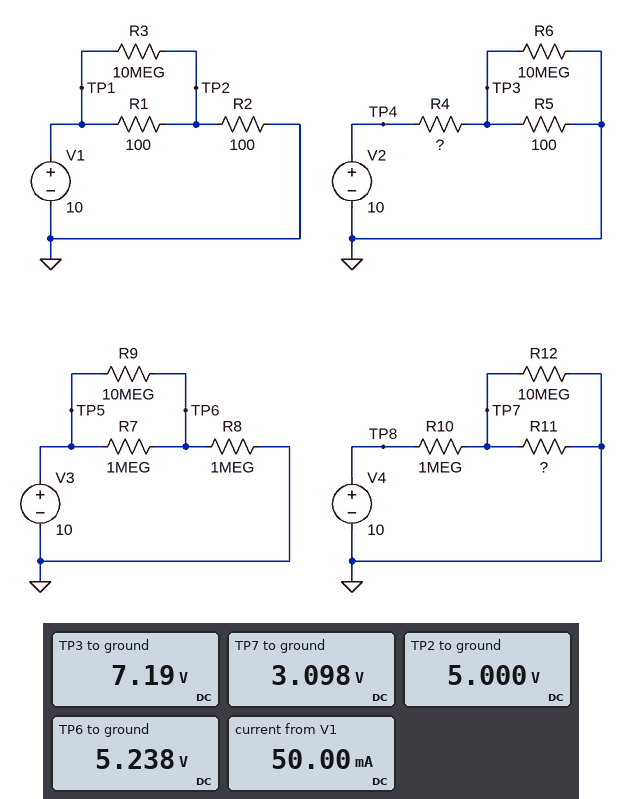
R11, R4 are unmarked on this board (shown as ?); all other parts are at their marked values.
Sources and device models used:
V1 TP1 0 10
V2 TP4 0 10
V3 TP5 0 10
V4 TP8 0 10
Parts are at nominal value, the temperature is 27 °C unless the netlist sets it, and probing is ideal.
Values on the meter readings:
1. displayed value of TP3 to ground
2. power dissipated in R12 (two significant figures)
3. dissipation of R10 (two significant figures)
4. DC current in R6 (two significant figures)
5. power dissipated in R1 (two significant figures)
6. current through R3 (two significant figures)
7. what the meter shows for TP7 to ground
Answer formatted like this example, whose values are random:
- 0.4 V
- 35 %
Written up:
- 7.19 V
- 960 nW
- 48 µW
- 720 nA
- 250 mW
- 500 nA
- 3.098 V
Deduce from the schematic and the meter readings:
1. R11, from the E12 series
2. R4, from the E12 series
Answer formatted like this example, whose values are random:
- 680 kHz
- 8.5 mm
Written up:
- 470 kΩ
- 39 Ω
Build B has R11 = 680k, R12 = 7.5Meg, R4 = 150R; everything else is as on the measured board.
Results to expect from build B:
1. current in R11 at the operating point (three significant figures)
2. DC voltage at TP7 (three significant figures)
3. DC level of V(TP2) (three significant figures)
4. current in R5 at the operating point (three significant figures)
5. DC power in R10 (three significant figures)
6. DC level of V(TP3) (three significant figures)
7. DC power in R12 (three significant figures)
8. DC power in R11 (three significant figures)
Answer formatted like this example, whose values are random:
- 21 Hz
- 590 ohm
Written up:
- 5.65 µA
- 3.84 V
- 5.00 V
- 40.0 mA
- 37.9 µW
- 4.00 V
- 1.97 µW
- 21.7 µW
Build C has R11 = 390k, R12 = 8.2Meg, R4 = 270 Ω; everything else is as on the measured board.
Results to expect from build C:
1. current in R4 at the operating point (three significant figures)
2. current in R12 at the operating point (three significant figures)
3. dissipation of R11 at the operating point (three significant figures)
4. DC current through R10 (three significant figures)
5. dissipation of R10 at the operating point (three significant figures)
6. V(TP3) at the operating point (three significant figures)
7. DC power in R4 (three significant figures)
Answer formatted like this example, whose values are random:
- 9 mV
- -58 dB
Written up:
- 27.0 mA
- 331 nA
- 18.9 µW
- 7.29 µA
- 53.1 µW
- 2.70 V
- 197 mW
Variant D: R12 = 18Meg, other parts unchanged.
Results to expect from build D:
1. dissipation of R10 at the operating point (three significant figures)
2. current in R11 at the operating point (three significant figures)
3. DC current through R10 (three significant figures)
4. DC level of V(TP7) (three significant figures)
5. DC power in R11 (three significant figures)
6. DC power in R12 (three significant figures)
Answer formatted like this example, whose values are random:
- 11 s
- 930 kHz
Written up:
- 47.0 µW
- 6.68 µA
- 6.86 µA
- 3.14 V
- 21.0 µW
- 548 nW
